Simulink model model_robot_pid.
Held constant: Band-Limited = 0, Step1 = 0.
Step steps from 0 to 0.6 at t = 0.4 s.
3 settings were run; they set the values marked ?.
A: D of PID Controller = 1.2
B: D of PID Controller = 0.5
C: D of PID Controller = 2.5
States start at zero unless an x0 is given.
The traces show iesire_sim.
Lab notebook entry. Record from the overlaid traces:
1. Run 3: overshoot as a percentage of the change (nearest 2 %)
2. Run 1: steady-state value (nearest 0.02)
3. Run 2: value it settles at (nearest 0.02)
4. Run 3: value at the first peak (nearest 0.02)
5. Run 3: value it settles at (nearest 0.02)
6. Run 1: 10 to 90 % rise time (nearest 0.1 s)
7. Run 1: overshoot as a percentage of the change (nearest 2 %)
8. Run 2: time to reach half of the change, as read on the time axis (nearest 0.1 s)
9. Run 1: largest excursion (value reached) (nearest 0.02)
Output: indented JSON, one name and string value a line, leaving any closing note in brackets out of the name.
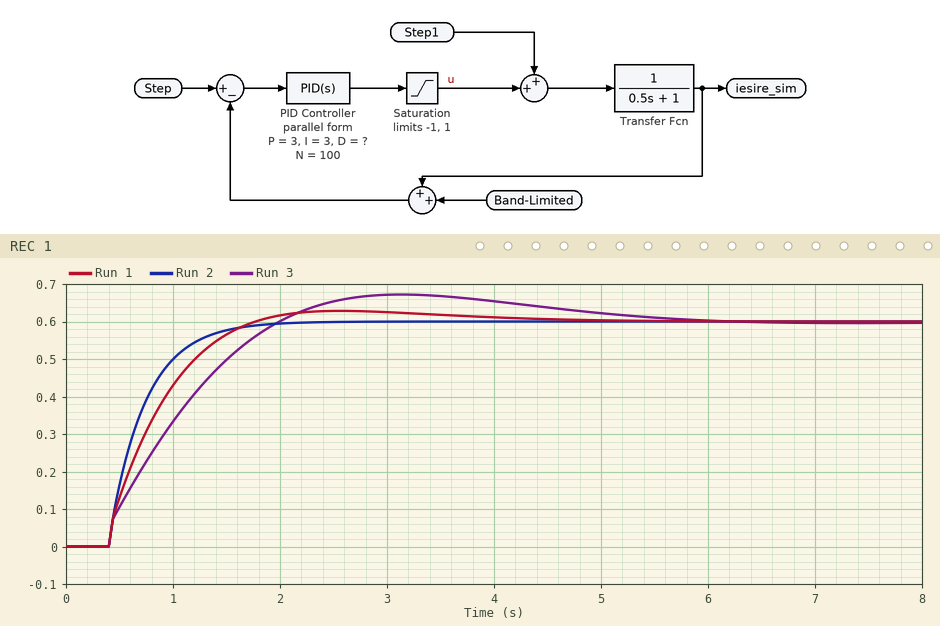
{
  "Run 3: overshoot as a percentage of the change": "12 %",
  "Run 1: steady-state value": "0.60",
  "Run 2: value it settles at": "0.60",
  "Run 3: value at the first peak": "0.68",
  "Run 3: value it settles at": "0.60",
  "Run 1: 10 to 90 % rise time": "0.9 s",
  "Run 1: overshoot as a percentage of the change": "4 %",
  "Run 2: time to reach half of the change, as read on the time axis": "0.6 s",
  "Run 1: largest excursion (value reached)": "0.62"
}
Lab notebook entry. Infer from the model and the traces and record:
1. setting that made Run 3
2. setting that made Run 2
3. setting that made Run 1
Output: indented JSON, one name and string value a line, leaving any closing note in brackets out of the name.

{
  "setting that made Run 3": "C",
  "setting that made Run 2": "B",
  "setting that made Run 1": "A"
}
